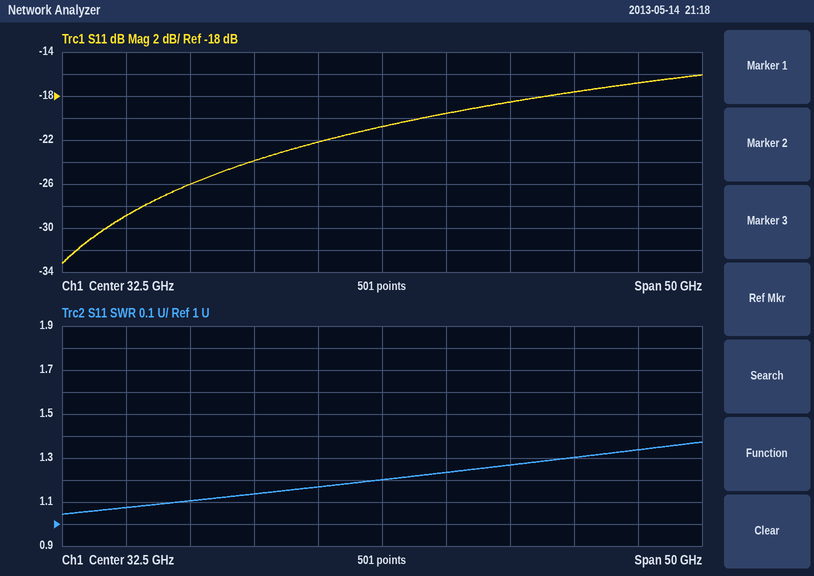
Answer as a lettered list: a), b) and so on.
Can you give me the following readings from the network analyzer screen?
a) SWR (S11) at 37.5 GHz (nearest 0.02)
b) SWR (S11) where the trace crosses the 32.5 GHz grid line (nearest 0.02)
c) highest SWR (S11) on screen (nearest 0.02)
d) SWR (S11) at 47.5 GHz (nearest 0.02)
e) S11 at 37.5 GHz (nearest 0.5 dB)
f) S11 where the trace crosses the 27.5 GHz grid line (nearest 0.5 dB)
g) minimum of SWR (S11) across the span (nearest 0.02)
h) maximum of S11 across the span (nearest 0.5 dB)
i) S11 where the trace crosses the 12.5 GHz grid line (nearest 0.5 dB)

a) 1.24
b) 1.20
c) 1.38
d) 1.30
e) -19.5 dB
f) -22.0 dB
g) 1.04
h) -16.0 dB
i) -29.0 dB
